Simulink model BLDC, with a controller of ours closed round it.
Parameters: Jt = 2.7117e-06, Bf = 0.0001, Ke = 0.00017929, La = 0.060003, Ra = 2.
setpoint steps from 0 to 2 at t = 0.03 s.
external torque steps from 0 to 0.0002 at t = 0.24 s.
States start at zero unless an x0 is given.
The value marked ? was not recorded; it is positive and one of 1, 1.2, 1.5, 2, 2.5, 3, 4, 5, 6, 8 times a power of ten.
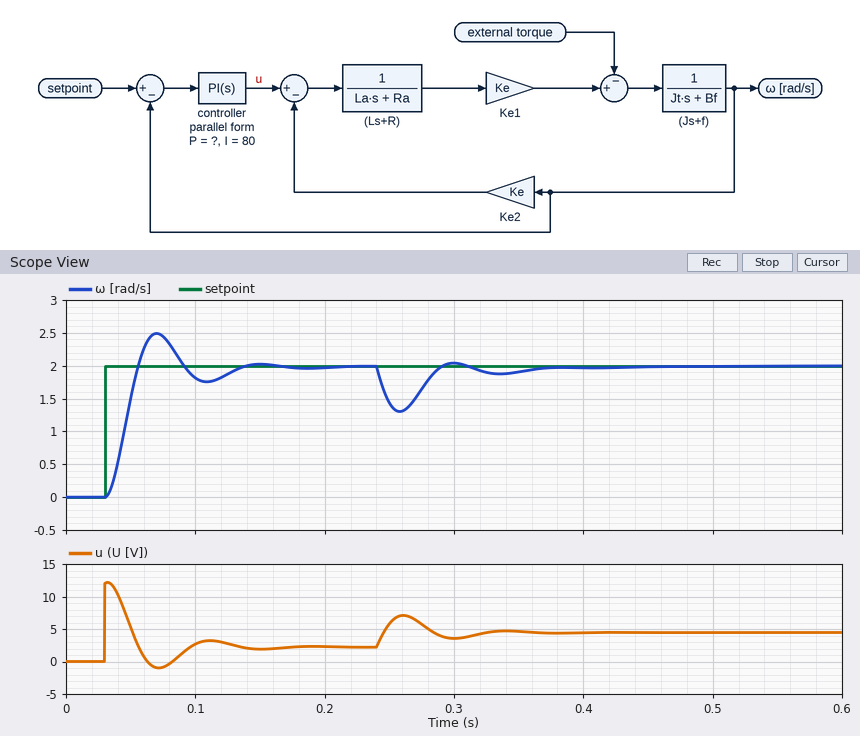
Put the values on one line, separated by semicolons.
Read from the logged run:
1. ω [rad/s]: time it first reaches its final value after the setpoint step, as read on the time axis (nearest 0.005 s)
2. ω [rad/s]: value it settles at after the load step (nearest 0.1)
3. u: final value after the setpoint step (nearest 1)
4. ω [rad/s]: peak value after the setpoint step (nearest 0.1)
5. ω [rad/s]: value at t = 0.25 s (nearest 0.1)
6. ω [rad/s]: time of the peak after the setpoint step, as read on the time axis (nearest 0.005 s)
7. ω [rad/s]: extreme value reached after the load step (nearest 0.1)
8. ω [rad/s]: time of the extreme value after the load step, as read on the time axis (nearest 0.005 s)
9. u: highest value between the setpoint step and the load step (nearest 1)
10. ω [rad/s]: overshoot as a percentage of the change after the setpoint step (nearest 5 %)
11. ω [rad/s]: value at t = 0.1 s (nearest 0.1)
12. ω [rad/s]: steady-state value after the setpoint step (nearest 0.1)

0.055 s; 2.0; 2; 2.5; 1.4; 0.070 s; 1.3; 0.260 s; 12; 25 %; 1.8; 2.0
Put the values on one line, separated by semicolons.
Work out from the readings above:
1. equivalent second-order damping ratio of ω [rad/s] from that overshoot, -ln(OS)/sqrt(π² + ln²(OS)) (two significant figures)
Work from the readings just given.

0.40
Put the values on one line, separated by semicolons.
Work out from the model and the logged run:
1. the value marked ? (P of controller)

6
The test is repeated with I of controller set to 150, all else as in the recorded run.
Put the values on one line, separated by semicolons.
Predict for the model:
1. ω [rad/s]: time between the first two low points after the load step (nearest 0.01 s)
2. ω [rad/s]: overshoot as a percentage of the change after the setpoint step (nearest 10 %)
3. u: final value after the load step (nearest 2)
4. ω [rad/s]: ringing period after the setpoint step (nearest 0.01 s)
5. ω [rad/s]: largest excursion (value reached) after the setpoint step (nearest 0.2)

0.08 s; 40 %; 4; 0.08 s; 2.8
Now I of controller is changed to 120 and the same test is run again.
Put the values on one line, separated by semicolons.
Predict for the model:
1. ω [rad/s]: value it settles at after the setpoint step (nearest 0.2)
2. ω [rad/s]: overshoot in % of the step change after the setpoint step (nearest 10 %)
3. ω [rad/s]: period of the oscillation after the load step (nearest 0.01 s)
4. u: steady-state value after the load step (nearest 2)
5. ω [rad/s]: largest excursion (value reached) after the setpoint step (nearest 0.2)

2.0; 30 %; 0.08 s; 4; 2.6
